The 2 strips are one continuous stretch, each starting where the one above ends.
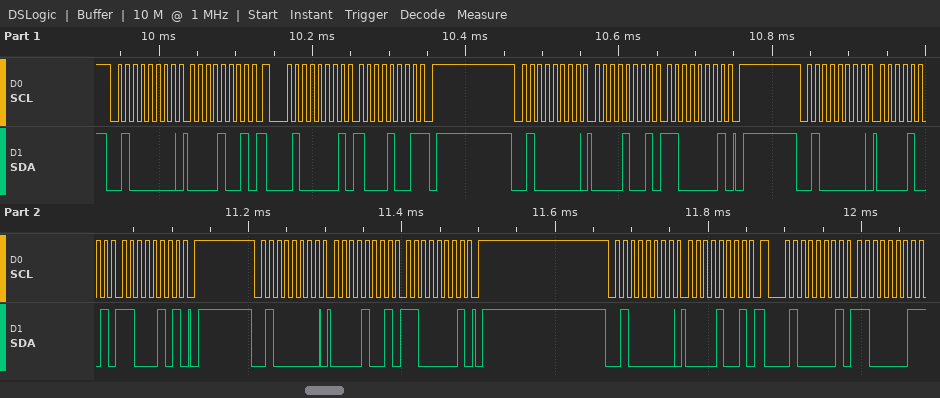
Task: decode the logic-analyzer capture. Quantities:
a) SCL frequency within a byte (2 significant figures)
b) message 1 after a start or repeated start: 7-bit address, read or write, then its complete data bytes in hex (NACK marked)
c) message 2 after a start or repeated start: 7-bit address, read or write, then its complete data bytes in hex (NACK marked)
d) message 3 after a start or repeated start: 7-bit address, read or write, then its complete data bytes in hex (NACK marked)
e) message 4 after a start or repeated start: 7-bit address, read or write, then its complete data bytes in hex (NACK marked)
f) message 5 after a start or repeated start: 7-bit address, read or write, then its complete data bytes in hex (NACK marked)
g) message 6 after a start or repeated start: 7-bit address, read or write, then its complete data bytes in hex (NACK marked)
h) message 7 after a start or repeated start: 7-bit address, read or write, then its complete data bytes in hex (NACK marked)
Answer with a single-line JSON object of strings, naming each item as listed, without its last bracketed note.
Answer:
{"SCL frequency within a byte": "100 kHz", "message 1 after a start or repeated start: 7-bit address, read or write, then its complete data bytes in hex": "0x20 write: 09", "message 2 after a start or repeated start: 7-bit address, read or write, then its complete data bytes in hex": "0x20 read: 89 NACK", "message 3 after a start or repeated start: 7-bit address, read or write, then its complete data bytes in hex": "0x20 write: 09 C1", "message 4 after a start or repeated start: 7-bit address, read or write, then its complete data bytes in hex": "0x20 write: 09 C5", "message 5 after a start or repeated start: 7-bit address, read or write, then its complete data bytes in hex": "0x20 write: 09 C1", "message 6 after a start or repeated start: 7-bit address, read or write, then its complete data bytes in hex": "0x20 write: 09", "message 7 after a start or repeated start: 7-bit address, read or write, then its complete data bytes in hex": "0x20 read: C1 NACK"}
